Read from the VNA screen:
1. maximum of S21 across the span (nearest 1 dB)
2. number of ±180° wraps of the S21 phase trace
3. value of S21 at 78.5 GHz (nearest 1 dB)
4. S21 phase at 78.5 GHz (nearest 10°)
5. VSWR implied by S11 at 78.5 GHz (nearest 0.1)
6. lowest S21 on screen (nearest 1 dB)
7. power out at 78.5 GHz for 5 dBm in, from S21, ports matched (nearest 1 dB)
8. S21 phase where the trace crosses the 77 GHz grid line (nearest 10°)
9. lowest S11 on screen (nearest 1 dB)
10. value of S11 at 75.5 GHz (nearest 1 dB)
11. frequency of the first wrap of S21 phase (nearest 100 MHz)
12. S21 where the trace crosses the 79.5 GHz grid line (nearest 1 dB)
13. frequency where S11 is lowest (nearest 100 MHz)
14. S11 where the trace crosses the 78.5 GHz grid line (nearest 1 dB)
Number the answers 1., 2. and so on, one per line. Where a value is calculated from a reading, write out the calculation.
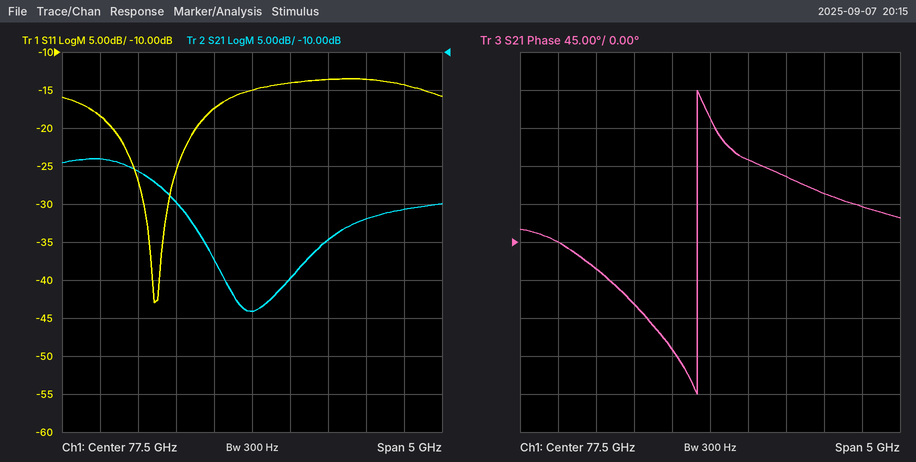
1. -24 dB
2. 1
3. -35 dB
4. 80°
5. |Γ| = 10^(-14/20) = 0.1995; VSWR = (1 + 0.1995)/(1 − 0.1995) ≈ 1.5
6. -44 dB
7. 5 dBm + (-35 dB) = -30 dBm
8. -130°
9. -43 dB
10. -18 dB
11. 77.3 GHz
12. -31 dB
13. 76.2 GHz
14. -14 dB
